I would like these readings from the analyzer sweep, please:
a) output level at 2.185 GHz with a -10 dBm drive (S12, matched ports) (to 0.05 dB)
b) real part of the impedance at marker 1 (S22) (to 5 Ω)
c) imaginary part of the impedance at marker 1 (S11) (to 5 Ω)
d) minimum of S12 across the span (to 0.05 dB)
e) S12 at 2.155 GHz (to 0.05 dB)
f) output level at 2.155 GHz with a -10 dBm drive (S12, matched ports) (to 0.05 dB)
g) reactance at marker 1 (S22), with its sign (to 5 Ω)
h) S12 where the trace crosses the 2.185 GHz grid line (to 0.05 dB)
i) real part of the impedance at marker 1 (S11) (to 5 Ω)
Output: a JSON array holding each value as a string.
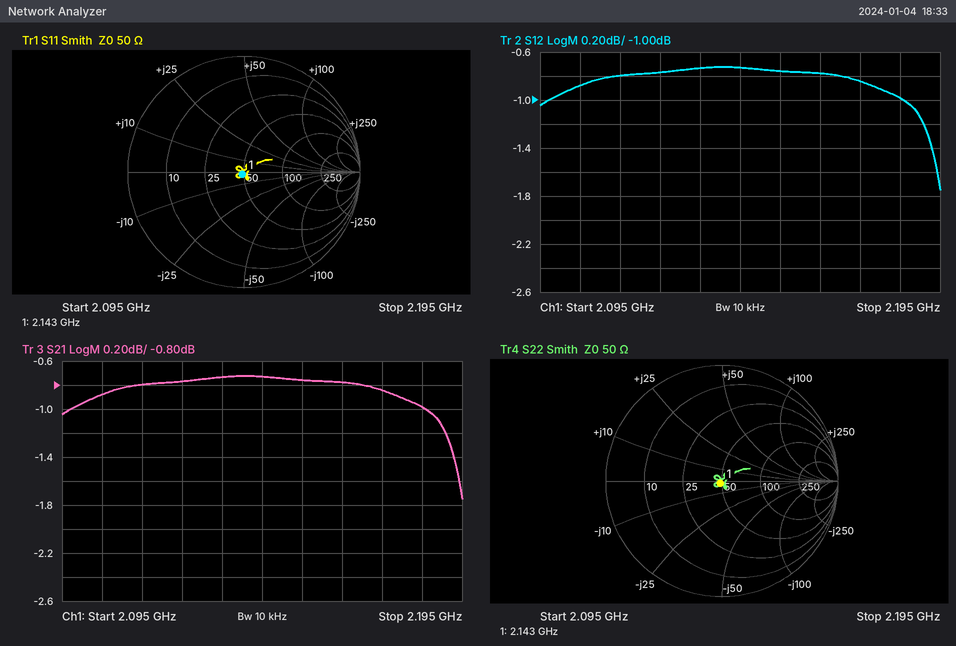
["-11.00 dBm", "50 Ω", "0 Ω", "-1.75 dB", "-0.75 dB", "-10.75 dBm", "0 Ω", "-1.00 dB", "50 Ω"]
